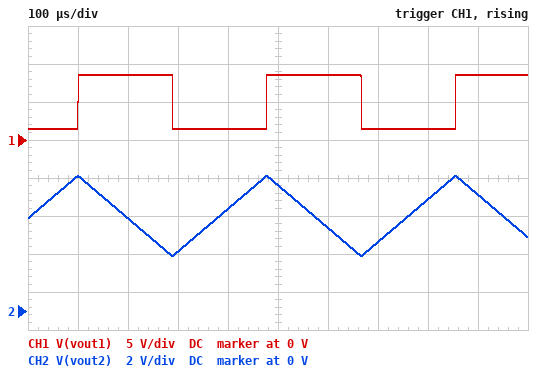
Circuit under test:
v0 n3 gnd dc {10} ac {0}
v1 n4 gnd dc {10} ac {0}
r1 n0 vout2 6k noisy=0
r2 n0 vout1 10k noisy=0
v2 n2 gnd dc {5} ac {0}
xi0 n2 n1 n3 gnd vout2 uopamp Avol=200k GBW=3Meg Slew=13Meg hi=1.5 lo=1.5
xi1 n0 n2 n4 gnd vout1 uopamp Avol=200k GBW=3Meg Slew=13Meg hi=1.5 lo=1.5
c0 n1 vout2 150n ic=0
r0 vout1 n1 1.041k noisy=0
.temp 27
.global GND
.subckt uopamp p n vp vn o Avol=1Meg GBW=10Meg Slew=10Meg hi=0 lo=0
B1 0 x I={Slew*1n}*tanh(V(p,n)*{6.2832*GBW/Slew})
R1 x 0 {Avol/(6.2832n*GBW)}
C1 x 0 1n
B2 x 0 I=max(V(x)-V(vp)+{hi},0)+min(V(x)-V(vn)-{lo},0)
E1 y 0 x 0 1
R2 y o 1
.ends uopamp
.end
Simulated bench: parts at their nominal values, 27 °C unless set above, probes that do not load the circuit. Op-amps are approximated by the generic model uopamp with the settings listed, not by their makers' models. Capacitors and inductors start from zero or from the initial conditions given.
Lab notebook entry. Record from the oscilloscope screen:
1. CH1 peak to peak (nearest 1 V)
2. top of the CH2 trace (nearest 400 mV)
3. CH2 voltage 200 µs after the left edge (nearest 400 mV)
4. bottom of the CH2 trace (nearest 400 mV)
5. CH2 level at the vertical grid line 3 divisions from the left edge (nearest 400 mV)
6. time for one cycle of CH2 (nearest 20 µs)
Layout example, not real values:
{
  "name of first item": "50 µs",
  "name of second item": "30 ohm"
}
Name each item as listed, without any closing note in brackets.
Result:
{
  "CH1 peak to peak": "7 V",
  "top of the CH2 trace": "7.2 V",
  "CH2 voltage 200 µs after the left edge": "4.8 V",
  "bottom of the CH2 trace": "2.8 V",
  "CH2 level at the vertical grid line 3 divisions from the left edge": "3.2 V",
  "time for one cycle of CH2": "380 µs"
}
